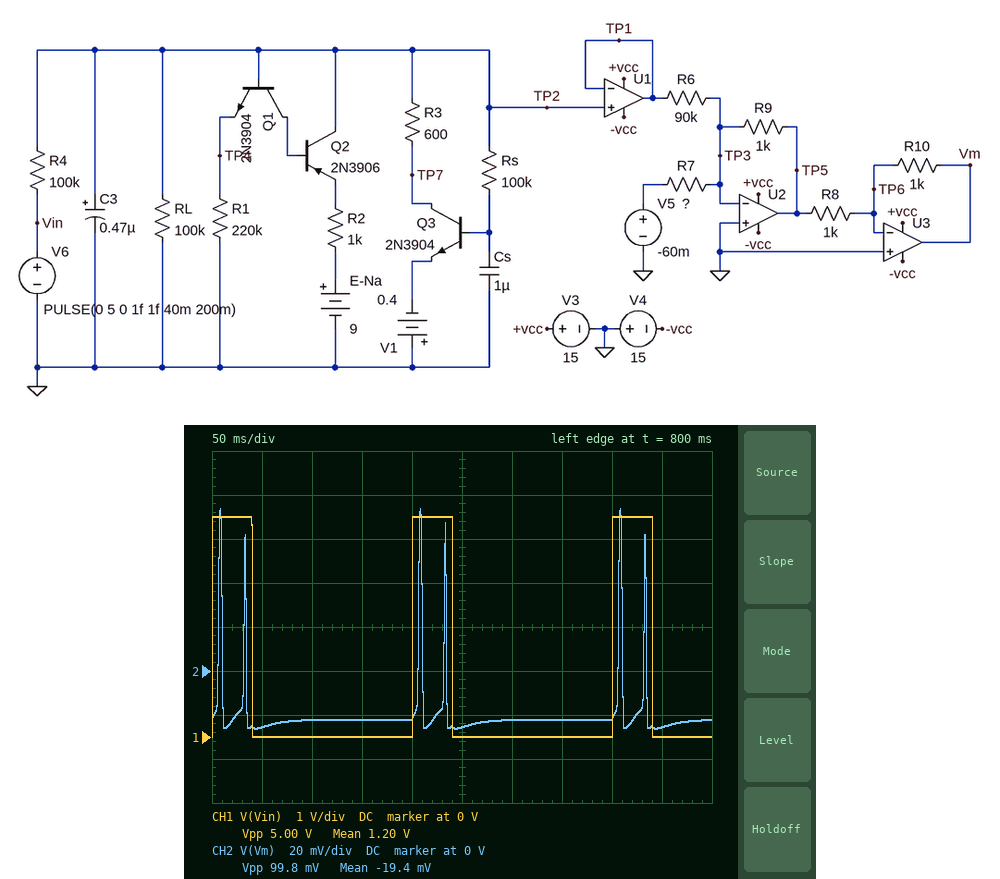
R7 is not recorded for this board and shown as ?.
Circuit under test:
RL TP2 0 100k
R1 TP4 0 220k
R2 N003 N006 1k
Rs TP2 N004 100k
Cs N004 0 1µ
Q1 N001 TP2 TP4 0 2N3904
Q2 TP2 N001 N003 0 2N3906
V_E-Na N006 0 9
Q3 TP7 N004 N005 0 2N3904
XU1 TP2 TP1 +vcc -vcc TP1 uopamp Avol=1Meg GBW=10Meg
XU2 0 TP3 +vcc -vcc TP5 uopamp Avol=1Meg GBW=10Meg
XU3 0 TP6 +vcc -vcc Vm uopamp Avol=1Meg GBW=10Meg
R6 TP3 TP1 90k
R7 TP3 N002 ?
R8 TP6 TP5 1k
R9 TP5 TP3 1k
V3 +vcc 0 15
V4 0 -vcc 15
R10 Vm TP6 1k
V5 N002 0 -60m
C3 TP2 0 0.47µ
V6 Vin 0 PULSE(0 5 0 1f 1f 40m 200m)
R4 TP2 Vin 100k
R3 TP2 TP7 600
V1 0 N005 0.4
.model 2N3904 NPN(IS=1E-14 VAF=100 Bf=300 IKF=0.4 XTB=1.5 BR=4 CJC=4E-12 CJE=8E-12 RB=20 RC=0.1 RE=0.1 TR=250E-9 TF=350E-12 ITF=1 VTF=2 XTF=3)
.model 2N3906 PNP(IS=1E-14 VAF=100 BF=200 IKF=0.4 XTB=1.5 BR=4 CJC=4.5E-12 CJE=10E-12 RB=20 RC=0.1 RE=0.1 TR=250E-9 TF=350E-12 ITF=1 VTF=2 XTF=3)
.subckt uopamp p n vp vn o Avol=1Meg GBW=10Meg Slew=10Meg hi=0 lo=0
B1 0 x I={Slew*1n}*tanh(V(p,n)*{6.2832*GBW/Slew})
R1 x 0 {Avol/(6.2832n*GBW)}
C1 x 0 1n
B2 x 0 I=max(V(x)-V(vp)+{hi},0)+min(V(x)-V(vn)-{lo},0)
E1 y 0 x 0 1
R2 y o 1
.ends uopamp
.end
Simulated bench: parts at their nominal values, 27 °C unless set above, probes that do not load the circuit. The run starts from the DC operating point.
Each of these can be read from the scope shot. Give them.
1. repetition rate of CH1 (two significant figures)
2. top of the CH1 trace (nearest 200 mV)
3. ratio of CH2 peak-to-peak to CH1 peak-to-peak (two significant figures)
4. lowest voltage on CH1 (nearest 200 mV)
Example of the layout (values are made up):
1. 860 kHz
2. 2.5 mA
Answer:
1. 5.0 Hz
2. 5.0 V
3. 0.020
4. 0 V
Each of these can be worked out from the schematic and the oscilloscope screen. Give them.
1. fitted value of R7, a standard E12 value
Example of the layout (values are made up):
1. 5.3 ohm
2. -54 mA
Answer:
1. 2.7 kΩ
